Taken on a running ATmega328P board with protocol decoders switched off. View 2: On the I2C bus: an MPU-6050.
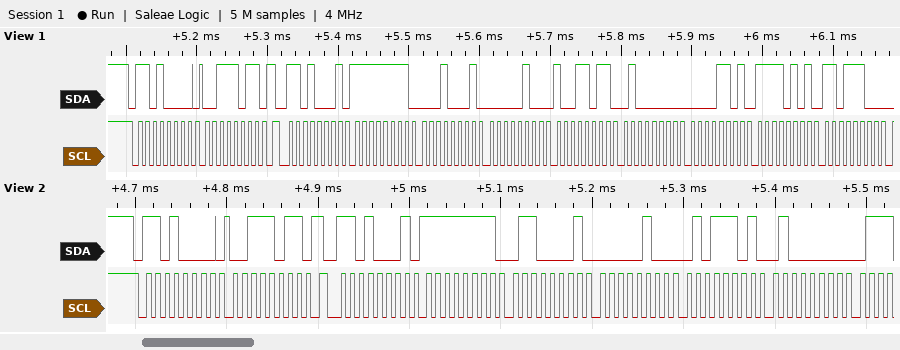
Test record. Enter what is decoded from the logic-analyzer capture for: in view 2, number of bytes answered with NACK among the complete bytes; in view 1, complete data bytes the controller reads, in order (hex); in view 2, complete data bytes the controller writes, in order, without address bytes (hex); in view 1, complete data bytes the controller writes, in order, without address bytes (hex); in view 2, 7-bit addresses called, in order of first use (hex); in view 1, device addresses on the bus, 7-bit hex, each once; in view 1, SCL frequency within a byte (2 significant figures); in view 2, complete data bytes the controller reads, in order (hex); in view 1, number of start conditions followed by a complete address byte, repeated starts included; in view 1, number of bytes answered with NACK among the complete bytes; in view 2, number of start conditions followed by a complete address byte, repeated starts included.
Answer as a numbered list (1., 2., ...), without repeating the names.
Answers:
1. 0
2. FF 11 04 9B 40 0D F5 DC
3. 3B
4. 3B
5. 0x68
6. 0x68
7. 100 kHz
8. FF 61 04 5D 40
9. 2
10. 0
11. 2
